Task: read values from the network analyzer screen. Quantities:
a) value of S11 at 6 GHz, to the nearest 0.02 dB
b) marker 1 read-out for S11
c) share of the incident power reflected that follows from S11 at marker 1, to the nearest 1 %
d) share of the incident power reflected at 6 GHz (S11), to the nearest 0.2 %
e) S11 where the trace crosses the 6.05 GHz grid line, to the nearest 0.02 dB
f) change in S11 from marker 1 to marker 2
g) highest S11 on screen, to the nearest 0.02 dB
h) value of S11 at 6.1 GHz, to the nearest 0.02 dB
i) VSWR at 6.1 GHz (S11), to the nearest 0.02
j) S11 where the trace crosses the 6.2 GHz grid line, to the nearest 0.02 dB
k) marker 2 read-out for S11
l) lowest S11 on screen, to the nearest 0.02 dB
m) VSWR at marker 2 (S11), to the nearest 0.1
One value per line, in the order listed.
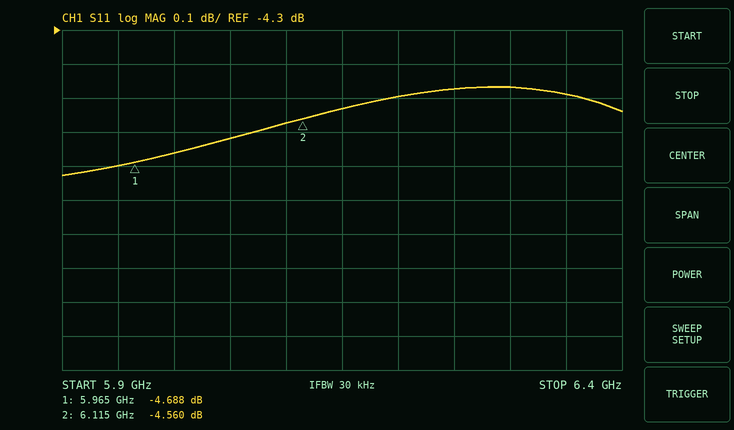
-4.66 dB
-4.688 dB
34 %
34.2 %
-4.62 dB
0.128 dB
-4.46 dB
-4.58 dB
3.88
-4.50 dB
-4.560 dB
-4.72 dB
3.9
